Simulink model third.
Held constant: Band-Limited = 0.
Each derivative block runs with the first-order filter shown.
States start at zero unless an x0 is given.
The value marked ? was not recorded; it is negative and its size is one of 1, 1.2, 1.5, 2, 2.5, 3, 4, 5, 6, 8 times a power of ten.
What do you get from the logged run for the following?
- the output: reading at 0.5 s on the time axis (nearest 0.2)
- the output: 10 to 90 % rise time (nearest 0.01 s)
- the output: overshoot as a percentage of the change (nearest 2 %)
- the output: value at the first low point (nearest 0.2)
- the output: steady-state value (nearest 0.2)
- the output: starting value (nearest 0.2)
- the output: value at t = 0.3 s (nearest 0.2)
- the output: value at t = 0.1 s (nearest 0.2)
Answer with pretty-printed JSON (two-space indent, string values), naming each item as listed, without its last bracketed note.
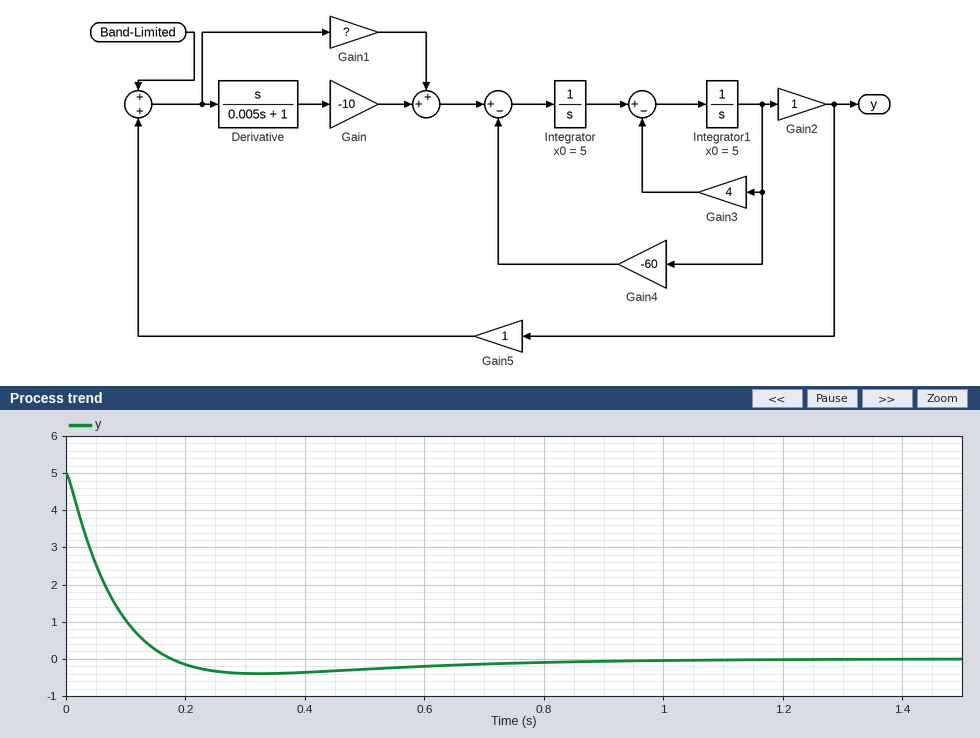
{
  "the output: reading at 0.5 s on the time axis": "-0.2",
  "the output: 10 to 90 % rise time": "0.12 s",
  "the output: overshoot as a percentage of the change": "8 %",
  "the output: value at the first low point": "-0.4",
  "the output: steady-state value": "0.0",
  "the output: starting value": "5.0",
  "the output: value at t = 0.3 s": "-0.4",
  "the output: value at t = 0.1 s": "1.0"
}
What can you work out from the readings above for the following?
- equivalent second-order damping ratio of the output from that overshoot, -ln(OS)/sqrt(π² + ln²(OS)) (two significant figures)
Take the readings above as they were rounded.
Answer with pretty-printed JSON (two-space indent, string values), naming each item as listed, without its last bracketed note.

{
  "equivalent second-order damping ratio of the output from that overshoot, -ln(OS)/sqrt(π² + ln²(OS))": "0.63"
}
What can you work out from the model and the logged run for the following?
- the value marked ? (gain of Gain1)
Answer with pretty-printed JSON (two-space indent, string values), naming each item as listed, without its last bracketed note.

{
  "the value marked ?": "-100"
}
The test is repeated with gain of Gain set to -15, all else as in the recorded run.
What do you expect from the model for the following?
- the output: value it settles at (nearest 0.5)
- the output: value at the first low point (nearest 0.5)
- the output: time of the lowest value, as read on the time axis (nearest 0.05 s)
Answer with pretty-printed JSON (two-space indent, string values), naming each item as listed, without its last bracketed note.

{
  "the output: value it settles at": "0.0",
  "the output: value at the first low point": "0.0",
  "the output: time of the lowest value, as read on the time axis": "0.30 s"
}
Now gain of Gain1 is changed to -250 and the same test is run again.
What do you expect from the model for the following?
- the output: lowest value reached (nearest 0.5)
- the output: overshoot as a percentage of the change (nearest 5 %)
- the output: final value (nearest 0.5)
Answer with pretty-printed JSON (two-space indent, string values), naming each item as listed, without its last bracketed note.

{
  "the output: lowest value reached": "-1.5",
  "the output: overshoot as a percentage of the change": "30 %",
  "the output: final value": "0.0"
}
